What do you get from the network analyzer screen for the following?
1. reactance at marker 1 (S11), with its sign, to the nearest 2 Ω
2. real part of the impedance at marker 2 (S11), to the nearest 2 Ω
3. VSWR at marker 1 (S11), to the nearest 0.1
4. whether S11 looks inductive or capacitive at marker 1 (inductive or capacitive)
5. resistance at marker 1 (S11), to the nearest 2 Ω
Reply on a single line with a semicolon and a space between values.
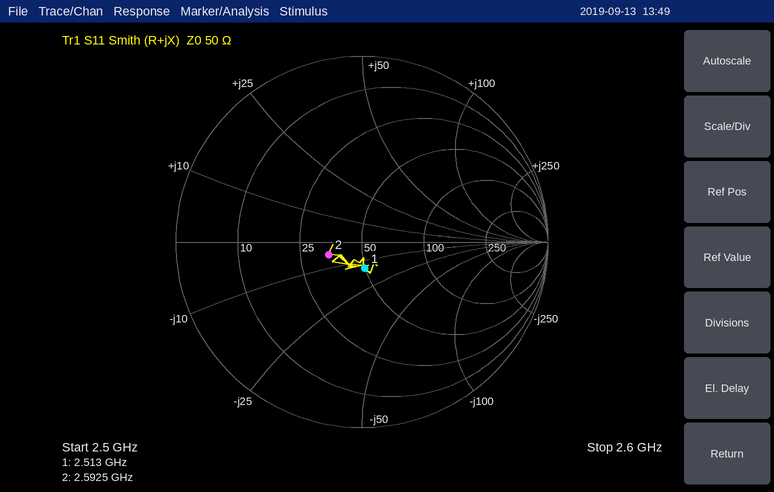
-14 Ω; 34 Ω; 1.3; capacitive; 50 Ω
